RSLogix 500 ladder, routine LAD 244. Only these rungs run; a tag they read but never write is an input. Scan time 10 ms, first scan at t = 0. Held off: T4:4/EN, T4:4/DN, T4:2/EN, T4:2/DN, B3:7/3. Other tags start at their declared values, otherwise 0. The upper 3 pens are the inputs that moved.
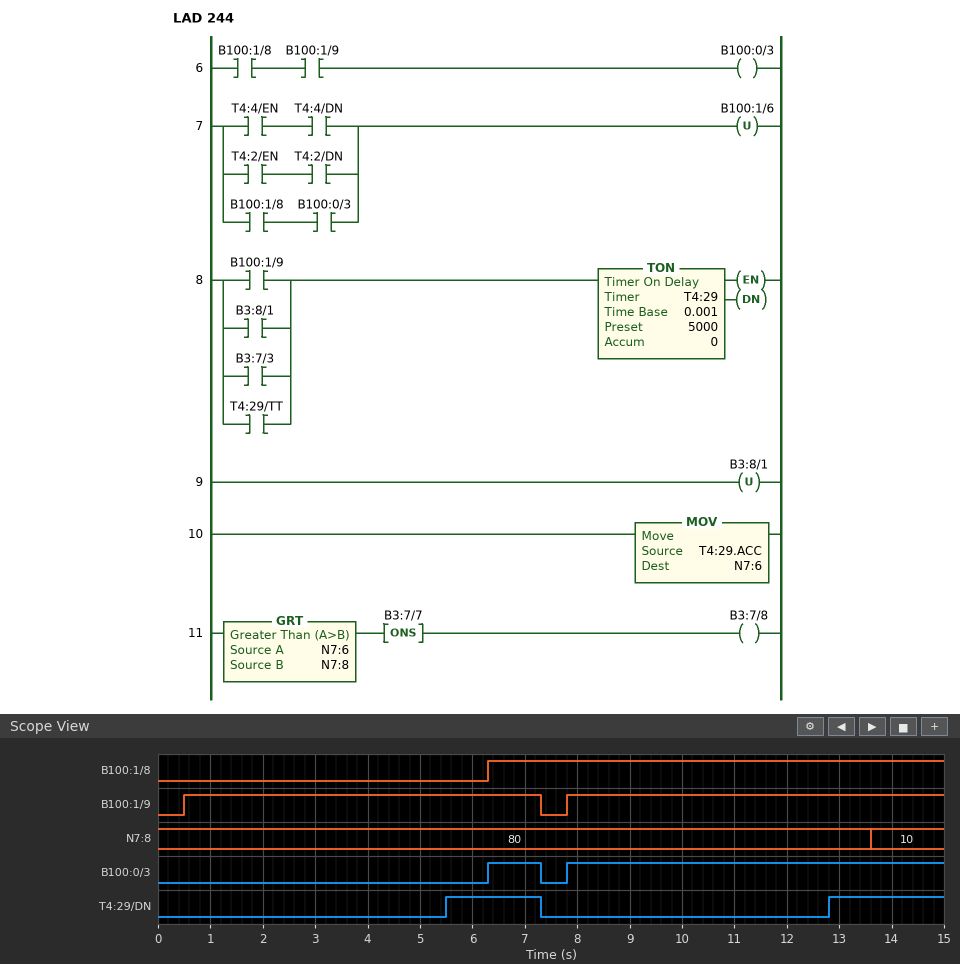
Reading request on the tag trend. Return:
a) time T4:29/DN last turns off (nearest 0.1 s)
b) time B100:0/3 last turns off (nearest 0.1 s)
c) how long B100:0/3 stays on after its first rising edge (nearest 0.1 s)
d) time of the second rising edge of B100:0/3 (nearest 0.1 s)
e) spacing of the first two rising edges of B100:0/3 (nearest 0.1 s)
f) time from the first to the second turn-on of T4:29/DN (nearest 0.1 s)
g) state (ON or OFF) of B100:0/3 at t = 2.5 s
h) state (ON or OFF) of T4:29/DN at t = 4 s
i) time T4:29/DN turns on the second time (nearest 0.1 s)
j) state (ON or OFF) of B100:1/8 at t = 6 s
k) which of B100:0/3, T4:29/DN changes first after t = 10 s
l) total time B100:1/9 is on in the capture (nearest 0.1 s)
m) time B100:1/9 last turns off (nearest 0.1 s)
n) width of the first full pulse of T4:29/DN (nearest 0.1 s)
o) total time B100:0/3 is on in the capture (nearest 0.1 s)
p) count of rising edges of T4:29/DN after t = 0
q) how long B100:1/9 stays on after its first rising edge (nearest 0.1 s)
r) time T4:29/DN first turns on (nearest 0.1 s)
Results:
7.3 s
7.3 s
1.0 s
7.8 s
1.5 s
7.3 s
OFF
OFF
12.8 s
OFF
T4:29/DN
14.0 s
7.3 s
1.8 s
8.2 s
2
6.8 s
5.5 s
